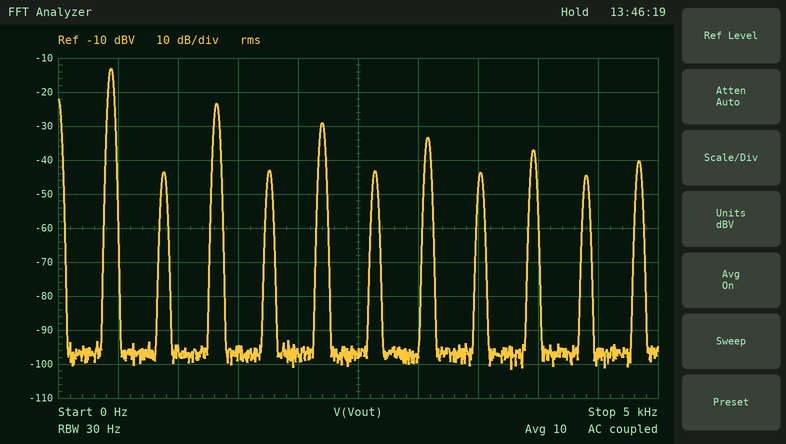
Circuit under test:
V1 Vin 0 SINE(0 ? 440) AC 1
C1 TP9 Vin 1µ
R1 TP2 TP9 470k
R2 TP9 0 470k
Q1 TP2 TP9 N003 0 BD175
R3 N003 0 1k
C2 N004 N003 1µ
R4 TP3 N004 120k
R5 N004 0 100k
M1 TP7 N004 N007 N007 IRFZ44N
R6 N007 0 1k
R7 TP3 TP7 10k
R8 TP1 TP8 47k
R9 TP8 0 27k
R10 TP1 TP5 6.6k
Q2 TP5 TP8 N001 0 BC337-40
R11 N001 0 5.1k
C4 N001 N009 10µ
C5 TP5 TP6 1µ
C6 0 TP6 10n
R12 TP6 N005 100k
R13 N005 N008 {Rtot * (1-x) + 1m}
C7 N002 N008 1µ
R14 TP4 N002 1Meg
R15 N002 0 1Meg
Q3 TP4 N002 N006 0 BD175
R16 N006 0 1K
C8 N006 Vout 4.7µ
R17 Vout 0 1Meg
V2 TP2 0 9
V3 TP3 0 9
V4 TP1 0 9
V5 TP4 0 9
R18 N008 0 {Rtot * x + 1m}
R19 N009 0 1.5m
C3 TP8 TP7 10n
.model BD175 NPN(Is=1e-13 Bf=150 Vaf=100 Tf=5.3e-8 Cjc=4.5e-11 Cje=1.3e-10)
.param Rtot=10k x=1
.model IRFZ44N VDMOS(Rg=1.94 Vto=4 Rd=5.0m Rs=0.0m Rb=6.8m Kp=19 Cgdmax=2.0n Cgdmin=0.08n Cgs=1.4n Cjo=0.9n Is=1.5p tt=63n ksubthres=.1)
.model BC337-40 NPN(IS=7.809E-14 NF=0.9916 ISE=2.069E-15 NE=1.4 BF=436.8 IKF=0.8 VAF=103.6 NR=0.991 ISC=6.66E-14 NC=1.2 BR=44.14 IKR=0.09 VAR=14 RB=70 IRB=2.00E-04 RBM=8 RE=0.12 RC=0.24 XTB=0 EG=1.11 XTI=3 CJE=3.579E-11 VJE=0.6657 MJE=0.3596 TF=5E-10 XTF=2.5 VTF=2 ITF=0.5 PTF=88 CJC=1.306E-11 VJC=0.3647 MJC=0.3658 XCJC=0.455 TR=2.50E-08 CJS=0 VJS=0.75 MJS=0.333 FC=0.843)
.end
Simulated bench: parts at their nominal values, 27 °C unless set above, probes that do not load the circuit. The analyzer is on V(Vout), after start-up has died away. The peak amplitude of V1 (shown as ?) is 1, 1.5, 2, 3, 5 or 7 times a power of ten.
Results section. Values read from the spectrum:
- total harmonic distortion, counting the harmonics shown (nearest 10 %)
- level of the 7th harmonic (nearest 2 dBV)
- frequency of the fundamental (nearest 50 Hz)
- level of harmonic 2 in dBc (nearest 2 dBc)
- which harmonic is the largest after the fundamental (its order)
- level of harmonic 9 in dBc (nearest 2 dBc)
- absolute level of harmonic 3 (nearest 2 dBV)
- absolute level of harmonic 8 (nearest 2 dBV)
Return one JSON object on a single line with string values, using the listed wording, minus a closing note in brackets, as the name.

{"total harmonic distortion, counting the harmonics shown": "40 %", "level of the 7th harmonic": "-34 dBV", "frequency of the fundamental": "450 Hz", "level of harmonic 2 in dBc": "-30 dBc", "which harmonic is the largest after the fundamental": "3", "level of harmonic 9 in dBc": "-24 dBc", "absolute level of harmonic 3": "-24 dBV", "absolute level of harmonic 8": "-44 dBV"}
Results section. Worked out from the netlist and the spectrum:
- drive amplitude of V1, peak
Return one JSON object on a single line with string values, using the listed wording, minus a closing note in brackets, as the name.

{"drive amplitude of V1, peak": "150 mV"}
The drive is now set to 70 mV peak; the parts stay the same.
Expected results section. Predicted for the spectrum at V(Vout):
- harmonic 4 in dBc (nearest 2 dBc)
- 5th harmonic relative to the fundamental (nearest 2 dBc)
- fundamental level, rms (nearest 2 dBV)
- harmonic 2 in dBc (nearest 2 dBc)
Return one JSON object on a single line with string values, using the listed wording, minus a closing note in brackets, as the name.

{"harmonic 4 in dBc": "-26 dBc", "5th harmonic relative to the fundamental": "-18 dBc", "fundamental level, rms": "-14 dBV", "harmonic 2 in dBc": "-24 dBc"}
